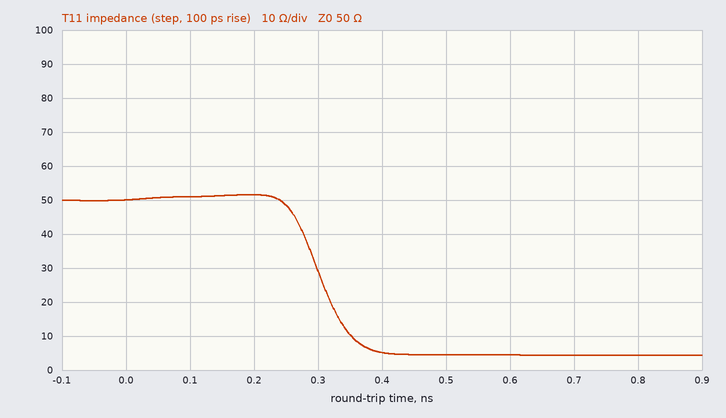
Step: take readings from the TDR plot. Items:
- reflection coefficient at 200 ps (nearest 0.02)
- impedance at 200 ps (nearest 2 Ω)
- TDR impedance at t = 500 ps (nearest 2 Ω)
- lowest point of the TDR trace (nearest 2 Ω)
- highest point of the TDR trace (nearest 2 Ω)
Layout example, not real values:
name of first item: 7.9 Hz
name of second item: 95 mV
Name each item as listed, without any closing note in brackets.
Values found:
reflection coefficient at 200 ps: +0.02
impedance at 200 ps: 52 Ω
TDR impedance at t = 500 ps: 4 Ω
lowest point of the TDR trace: 4 Ω
highest point of the TDR trace: 52 Ω
